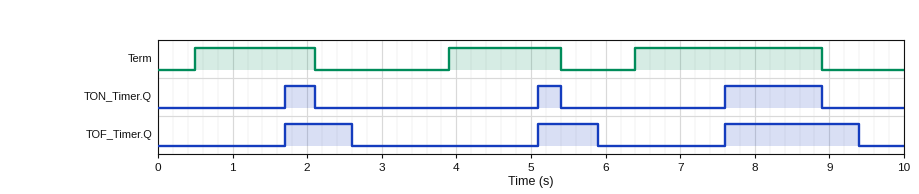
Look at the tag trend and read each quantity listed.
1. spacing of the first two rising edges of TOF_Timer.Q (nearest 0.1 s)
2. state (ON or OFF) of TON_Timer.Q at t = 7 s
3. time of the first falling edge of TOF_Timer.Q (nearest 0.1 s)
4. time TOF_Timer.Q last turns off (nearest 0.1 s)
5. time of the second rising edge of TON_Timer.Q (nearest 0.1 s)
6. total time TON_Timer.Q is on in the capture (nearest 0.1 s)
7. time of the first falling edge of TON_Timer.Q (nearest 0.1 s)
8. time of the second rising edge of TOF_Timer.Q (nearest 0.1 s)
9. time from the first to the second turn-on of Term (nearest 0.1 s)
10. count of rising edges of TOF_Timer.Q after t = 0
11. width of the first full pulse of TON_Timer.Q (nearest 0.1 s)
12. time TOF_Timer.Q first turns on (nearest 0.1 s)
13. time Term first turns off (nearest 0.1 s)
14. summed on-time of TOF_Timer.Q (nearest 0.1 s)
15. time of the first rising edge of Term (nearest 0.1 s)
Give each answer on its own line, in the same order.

3.4 s
OFF
2.6 s
9.4 s
5.1 s
2.0 s
2.1 s
5.1 s
3.4 s
3
0.4 s
1.7 s
2.1 s
3.5 s
0.5 s
